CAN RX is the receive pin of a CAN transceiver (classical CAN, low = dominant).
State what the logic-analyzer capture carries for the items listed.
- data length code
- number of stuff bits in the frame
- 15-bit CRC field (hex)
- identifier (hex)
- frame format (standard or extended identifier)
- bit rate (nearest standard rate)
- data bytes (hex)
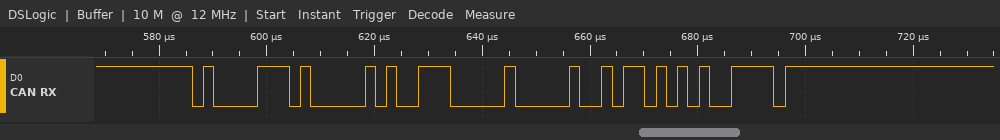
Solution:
2
3
0x5AA7
0x43A
standard
500 kbit/s
70 00
